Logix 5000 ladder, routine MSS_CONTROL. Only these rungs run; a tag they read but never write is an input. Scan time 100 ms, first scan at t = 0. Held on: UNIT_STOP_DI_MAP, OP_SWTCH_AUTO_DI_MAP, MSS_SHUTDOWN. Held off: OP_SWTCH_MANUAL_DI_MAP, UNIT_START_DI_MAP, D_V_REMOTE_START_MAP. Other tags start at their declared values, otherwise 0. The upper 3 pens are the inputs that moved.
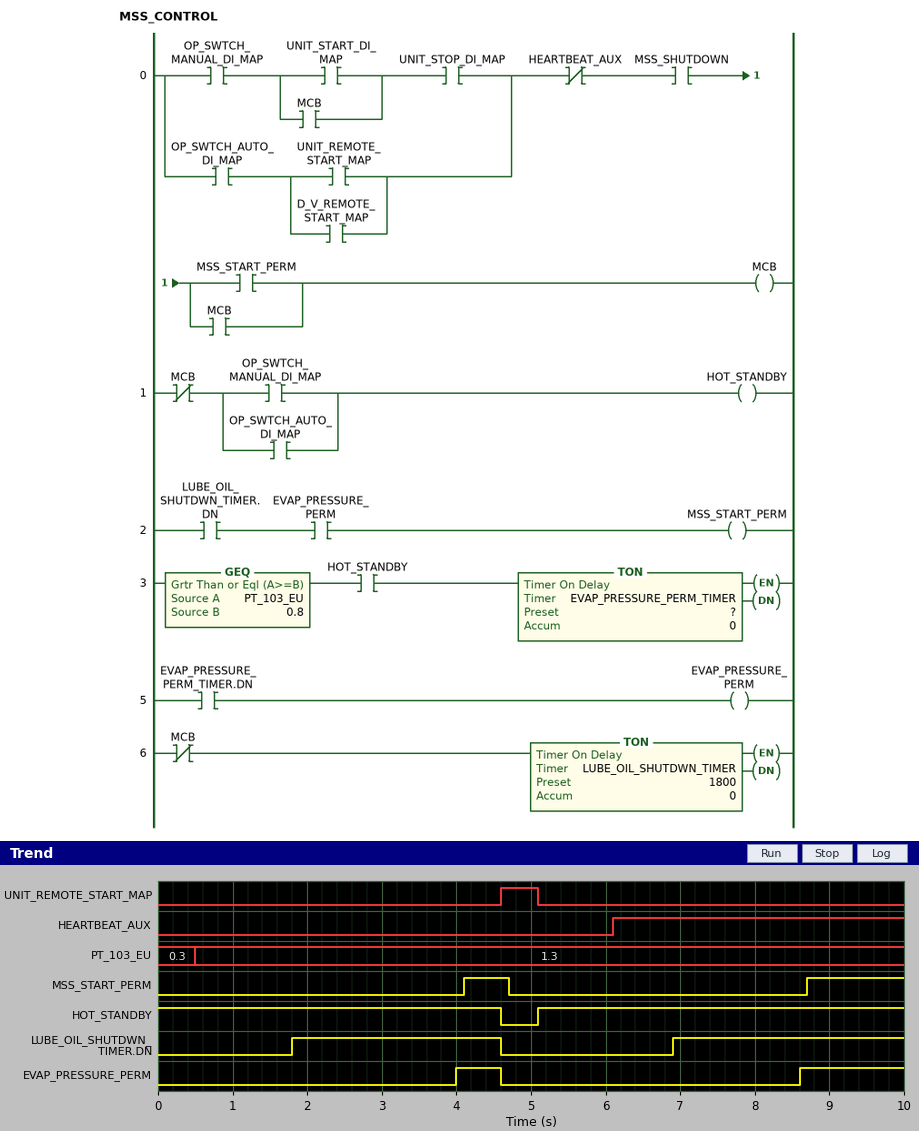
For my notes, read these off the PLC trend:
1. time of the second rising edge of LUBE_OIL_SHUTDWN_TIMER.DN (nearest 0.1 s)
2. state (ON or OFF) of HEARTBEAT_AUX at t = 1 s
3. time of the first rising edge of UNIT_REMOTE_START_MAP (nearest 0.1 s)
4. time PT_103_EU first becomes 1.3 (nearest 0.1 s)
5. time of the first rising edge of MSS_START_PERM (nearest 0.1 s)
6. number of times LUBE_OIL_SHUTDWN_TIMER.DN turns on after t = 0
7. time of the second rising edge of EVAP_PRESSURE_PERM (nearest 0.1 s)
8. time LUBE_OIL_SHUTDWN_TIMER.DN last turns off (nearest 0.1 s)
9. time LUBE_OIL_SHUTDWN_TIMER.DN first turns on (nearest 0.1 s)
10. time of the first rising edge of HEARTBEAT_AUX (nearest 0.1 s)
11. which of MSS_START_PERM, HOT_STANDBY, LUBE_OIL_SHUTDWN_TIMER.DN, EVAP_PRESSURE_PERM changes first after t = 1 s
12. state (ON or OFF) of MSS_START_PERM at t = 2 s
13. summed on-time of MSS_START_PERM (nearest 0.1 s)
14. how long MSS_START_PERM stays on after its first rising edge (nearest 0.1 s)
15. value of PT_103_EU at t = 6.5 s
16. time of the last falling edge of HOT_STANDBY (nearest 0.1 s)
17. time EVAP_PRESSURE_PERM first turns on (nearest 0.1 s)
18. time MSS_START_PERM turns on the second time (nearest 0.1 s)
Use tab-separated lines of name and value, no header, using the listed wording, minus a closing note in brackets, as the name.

time of the second rising edge of LUBE_OIL_SHUTDWN_TIMER.DN	6.9 s
state (ON or OFF) of HEARTBEAT_AUX at t = 1 s	OFF
time of the first rising edge of UNIT_REMOTE_START_MAP	4.6 s
time PT_103_EU first becomes 1.3	0.5 s
time of the first rising edge of MSS_START_PERM	4.1 s
number of times LUBE_OIL_SHUTDWN_TIMER.DN turns on after t = 0	2
time of the second rising edge of EVAP_PRESSURE_PERM	8.6 s
time LUBE_OIL_SHUTDWN_TIMER.DN last turns off	4.6 s
time LUBE_OIL_SHUTDWN_TIMER.DN first turns on	1.8 s
time of the first rising edge of HEARTBEAT_AUX	6.1 s
which of MSS_START_PERM, HOT_STANDBY, LUBE_OIL_SHUTDWN_TIMER.DN, EVAP_PRESSURE_PERM changes first after t = 1 s	LUBE_OIL_SHUTDWN_TIMER.DN
state (ON or OFF) of MSS_START_PERM at t = 2 s	OFF
summed on-time of MSS_START_PERM	1.9 s
how long MSS_START_PERM stays on after its first rising edge	0.6 s
value of PT_103_EU at t = 6.5 s	1.3
time of the last falling edge of HOT_STANDBY	4.6 s
time EVAP_PRESSURE_PERM first turns on	4.0 s
time MSS_START_PERM turns on the second time	8.7 s
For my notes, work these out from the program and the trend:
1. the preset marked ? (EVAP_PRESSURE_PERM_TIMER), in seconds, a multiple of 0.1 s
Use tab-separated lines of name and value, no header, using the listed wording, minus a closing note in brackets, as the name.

the preset marked ? (EVAP_PRESSURE_PERM_TIMER), in seconds, a multiple of 0.1 s	3.5 s
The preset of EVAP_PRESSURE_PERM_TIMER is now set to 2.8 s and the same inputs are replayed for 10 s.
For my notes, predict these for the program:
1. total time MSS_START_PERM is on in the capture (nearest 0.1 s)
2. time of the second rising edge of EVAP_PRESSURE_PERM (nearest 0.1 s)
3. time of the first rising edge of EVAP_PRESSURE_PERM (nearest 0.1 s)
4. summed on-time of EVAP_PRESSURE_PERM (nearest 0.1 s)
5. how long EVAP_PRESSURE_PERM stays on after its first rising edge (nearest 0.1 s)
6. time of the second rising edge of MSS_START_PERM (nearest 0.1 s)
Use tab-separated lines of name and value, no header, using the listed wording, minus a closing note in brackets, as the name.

total time MSS_START_PERM is on in the capture	3.3 s
time of the second rising edge of EVAP_PRESSURE_PERM	7.9 s
time of the first rising edge of EVAP_PRESSURE_PERM	3.3 s
summed on-time of EVAP_PRESSURE_PERM	3.4 s
how long EVAP_PRESSURE_PERM stays on after its first rising edge	1.3 s
time of the second rising edge of MSS_START_PERM	8.0 s
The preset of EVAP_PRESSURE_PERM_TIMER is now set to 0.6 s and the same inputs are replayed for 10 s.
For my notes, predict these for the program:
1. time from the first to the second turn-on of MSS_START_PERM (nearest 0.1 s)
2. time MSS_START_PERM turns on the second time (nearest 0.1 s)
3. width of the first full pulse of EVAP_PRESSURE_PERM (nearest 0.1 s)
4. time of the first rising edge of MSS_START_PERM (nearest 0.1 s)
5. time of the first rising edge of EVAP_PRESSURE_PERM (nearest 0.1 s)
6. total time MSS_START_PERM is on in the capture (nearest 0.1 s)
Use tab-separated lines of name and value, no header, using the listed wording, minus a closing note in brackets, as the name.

time from the first to the second turn-on of MSS_START_PERM	5.1 s
time MSS_START_PERM turns on the second time	7.0 s
width of the first full pulse of EVAP_PRESSURE_PERM	3.5 s
time of the first rising edge of MSS_START_PERM	1.9 s
time of the first rising edge of EVAP_PRESSURE_PERM	1.1 s
total time MSS_START_PERM is on in the capture	5.8 s
